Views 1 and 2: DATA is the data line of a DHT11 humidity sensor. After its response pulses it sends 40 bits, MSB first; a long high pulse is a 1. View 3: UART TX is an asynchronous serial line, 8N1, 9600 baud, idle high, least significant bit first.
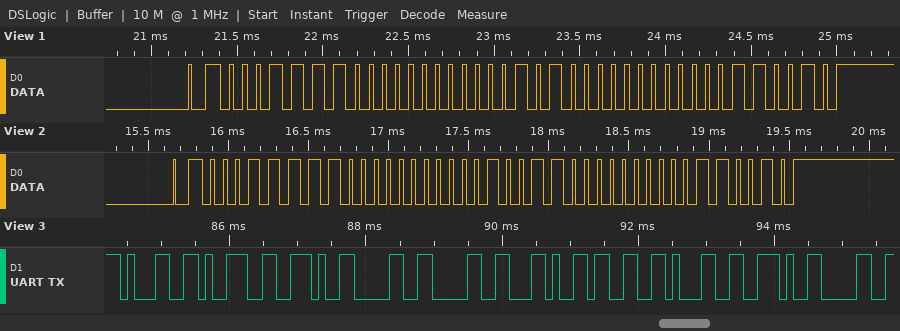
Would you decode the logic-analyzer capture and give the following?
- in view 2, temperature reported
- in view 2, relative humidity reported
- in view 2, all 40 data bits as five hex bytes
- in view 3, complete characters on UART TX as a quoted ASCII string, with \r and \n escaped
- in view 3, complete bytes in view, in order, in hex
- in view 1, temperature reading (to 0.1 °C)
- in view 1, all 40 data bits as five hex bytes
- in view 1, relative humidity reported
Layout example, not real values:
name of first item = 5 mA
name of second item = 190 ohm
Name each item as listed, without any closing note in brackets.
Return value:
in view 2, temperature reported = 19.0 °C
in view 2, relative humidity reported = 31 %
in view 2, all 40 data bits as five hex bytes = 1F 00 13 00 32
in view 3, complete characters on UART TX as a quoted ASCII string, with \r and \n escaped = "19.00,31.0"
in view 3, complete bytes in view, in order, in hex = 0x31 0x39 0x2E 0x30 0x30 0x2C 0x33 0x31 0x2E 0x30
in view 1, temperature reading = 20.0 °C
in view 1, all 40 data bits as five hex bytes = 1E 00 14 00 32
in view 1, relative humidity reported = 30 %
